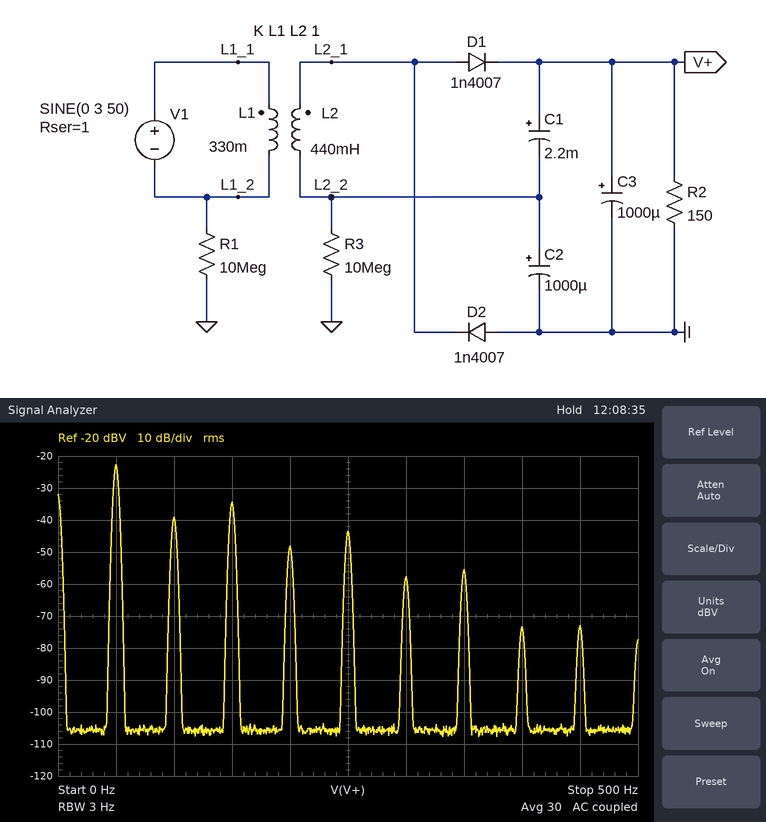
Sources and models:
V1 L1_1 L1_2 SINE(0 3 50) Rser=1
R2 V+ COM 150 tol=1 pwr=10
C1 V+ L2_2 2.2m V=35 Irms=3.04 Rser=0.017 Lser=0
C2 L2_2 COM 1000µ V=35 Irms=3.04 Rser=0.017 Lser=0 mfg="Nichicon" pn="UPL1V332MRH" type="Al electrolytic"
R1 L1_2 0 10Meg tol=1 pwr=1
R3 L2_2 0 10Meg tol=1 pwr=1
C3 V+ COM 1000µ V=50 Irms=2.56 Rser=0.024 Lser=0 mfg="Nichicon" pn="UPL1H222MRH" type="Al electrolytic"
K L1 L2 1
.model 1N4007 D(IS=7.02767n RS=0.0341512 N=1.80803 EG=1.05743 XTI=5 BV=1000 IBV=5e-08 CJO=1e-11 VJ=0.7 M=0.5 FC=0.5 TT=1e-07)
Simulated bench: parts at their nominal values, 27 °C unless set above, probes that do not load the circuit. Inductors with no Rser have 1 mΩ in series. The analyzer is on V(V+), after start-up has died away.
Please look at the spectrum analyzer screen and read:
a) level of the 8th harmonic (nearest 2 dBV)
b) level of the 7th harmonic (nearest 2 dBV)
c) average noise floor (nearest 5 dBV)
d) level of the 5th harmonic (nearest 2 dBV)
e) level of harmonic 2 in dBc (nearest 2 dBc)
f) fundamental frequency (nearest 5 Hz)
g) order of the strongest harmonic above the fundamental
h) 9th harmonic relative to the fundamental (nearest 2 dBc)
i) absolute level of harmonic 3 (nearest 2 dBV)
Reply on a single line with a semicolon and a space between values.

-74 dBV; -56 dBV; -105 dBV; -44 dBV; -16 dBc; 50 Hz; 3; -50 dBc; -34 dBV
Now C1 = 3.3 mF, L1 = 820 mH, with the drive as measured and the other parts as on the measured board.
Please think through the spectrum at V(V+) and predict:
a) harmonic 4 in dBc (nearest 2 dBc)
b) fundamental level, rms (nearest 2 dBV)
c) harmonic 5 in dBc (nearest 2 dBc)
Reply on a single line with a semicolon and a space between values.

-24 dBc; -30 dBV; -18 dBc
